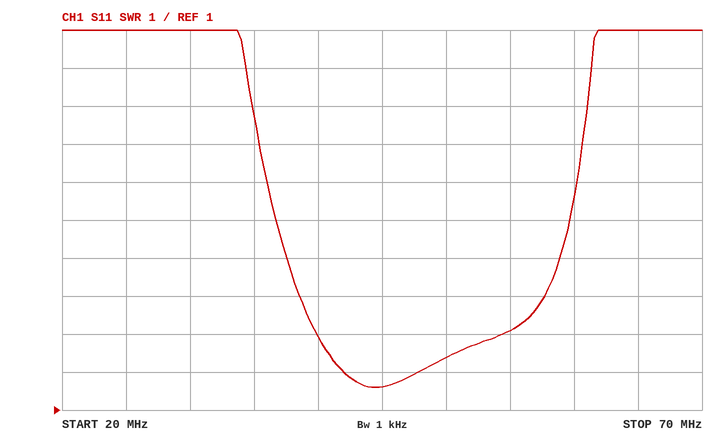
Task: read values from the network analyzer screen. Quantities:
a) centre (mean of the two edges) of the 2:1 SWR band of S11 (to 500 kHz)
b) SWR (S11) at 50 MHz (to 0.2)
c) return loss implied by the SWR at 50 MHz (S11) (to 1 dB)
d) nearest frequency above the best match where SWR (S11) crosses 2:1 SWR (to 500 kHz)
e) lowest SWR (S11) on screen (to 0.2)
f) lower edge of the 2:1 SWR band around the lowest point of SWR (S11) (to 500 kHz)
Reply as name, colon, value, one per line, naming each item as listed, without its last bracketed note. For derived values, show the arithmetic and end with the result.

centre (mean of the two edges) of the 2:1 SWR band of S11: 45.0 MHz
SWR (S11) at 50 MHz: 2.4
return loss implied by the SWR at 50 MHz (S11): −20 log10((2.4 − 1)/(2.4 + 1)) ≈ 8 dB
nearest frequency above the best match where SWR (S11) crosses 2:1 SWR: 48.0 MHz
lowest SWR (S11) on screen: 1.6
lower edge of the 2:1 SWR band around the lowest point of SWR (S11): 42.0 MHz
